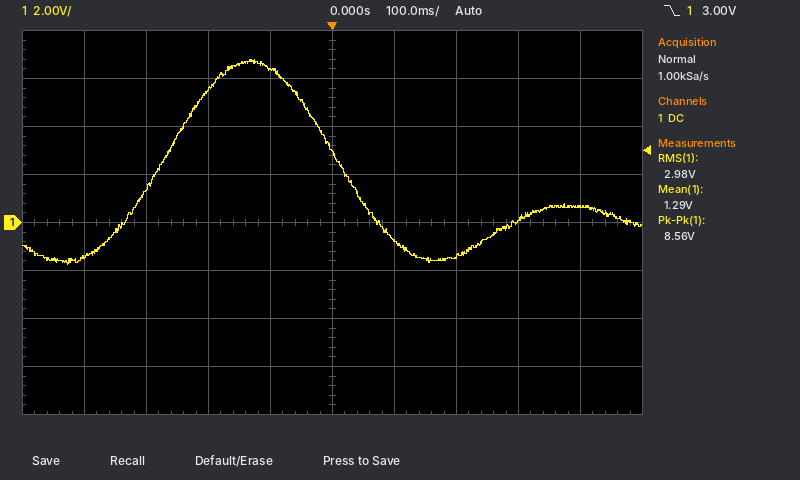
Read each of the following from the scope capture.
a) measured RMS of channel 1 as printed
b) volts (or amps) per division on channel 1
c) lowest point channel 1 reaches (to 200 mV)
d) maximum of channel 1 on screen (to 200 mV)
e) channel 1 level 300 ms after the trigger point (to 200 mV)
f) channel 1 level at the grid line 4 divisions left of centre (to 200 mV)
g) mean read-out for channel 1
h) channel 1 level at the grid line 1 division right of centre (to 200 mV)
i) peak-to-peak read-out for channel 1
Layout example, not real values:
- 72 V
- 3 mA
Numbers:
- 2.98 V
- 2 V
- -1.8 V
- 6.8 V
- 0.0 V
- -1.4 V
- 1.29 V
- -800 mV
- 8.56 V
